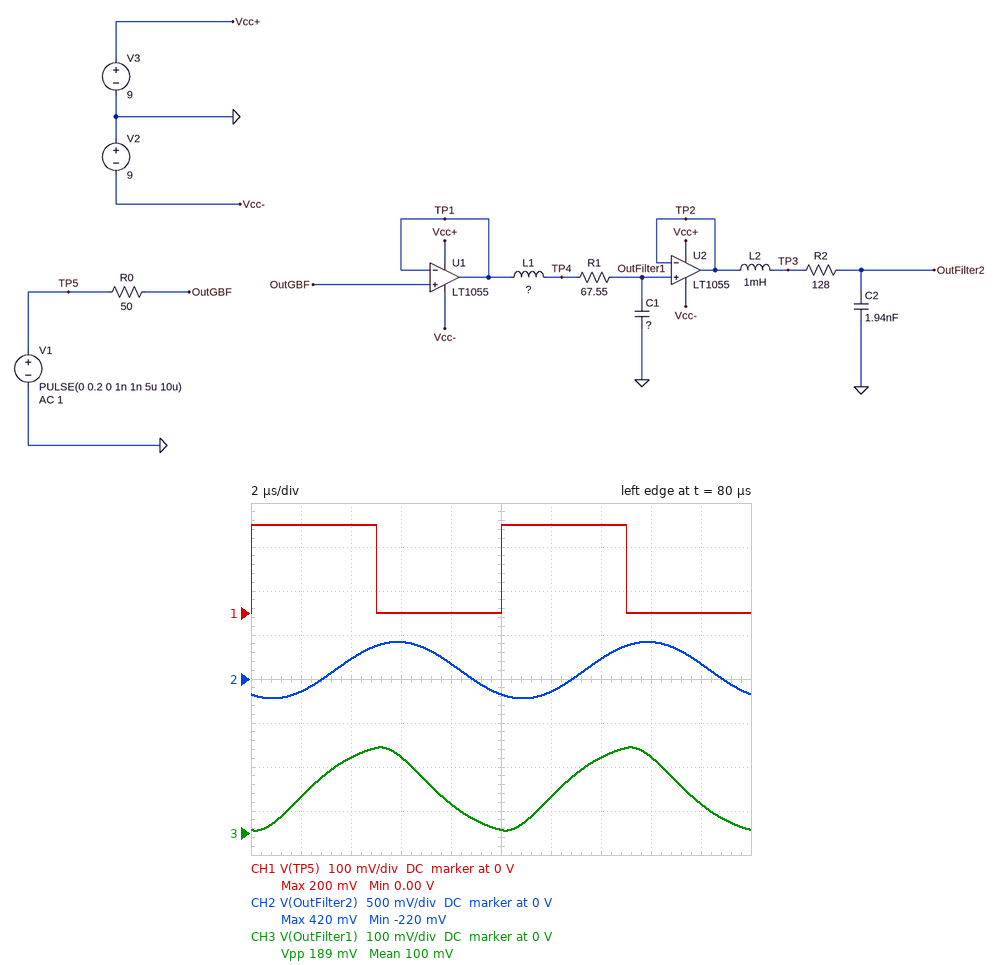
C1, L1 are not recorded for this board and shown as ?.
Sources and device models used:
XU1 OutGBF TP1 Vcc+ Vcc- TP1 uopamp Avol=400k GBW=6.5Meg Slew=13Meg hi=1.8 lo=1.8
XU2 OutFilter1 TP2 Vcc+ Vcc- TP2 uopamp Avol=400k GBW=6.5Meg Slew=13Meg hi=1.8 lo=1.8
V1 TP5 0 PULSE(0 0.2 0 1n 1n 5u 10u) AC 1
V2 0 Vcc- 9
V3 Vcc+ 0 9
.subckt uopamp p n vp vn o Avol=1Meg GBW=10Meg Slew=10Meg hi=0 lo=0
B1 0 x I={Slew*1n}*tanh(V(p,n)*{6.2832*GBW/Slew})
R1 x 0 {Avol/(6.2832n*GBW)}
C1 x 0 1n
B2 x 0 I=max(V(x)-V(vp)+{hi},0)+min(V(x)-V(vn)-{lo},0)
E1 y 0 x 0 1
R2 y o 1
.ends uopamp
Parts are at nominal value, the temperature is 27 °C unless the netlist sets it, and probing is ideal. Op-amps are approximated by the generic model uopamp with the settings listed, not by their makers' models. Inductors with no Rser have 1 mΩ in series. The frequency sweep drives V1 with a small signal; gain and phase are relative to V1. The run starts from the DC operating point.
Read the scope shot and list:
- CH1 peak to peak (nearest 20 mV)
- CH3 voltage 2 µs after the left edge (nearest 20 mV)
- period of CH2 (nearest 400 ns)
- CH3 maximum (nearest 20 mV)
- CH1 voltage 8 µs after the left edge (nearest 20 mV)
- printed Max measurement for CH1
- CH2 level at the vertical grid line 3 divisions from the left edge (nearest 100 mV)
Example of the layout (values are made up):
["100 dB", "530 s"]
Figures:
["200 mV", "80 mV", "10.0 µs", "200 mV", "0 V", "200 mV", "400 mV"]
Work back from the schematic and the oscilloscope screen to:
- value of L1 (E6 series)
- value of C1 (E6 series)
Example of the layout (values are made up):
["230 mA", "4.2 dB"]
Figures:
["68 µH", "33 nF"]
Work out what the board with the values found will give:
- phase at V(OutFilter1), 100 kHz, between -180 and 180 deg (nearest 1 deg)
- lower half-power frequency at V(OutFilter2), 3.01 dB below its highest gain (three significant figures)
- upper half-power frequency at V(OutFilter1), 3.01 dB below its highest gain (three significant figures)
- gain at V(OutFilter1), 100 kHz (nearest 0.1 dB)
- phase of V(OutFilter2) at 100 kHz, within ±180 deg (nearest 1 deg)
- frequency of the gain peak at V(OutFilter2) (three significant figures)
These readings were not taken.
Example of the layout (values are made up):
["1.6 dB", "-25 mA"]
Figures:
["-86 deg", "99.8 kHz", "101 kHz", "-3.0 dB", "-121 deg", "112 kHz"]
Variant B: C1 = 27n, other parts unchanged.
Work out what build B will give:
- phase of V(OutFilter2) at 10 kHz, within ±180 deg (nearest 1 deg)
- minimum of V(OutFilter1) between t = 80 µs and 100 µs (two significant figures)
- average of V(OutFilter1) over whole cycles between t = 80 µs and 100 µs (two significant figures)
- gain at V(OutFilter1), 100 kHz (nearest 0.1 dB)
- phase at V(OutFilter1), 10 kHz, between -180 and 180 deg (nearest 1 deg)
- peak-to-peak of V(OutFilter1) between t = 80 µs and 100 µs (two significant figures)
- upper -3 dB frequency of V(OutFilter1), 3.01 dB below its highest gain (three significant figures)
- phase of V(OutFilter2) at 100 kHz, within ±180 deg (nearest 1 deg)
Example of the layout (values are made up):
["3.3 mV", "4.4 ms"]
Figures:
["-8 deg", "-9.4 mV", "100 mV", "-1.4 dB", "-7 deg", "220 mV", "123 kHz", "-112 deg"]
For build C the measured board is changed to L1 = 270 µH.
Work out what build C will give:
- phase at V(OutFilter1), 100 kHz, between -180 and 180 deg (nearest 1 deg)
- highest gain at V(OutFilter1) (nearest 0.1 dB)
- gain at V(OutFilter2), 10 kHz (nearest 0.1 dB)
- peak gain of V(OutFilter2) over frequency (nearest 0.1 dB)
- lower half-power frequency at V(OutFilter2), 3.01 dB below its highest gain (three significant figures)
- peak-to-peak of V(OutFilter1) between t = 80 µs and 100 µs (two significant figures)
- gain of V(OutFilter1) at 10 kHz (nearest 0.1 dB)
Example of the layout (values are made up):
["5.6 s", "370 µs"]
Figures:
["-152 deg", "3.2 dB", "0.3 dB", "4.8 dB", "24.9 kHz", "88 mV", "0.2 dB"]
